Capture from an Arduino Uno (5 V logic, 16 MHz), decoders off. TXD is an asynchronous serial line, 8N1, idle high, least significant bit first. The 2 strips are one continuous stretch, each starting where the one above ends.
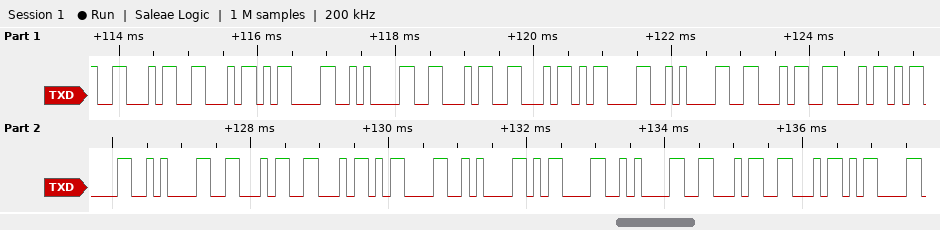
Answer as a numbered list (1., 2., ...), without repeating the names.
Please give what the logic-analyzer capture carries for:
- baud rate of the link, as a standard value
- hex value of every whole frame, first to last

1. 9600 baud
2. 46 46 0D 0A 46 46 0D 0A 46 46 0D 0A 46 46 0D 0A 0D 0A 46 46 0D
